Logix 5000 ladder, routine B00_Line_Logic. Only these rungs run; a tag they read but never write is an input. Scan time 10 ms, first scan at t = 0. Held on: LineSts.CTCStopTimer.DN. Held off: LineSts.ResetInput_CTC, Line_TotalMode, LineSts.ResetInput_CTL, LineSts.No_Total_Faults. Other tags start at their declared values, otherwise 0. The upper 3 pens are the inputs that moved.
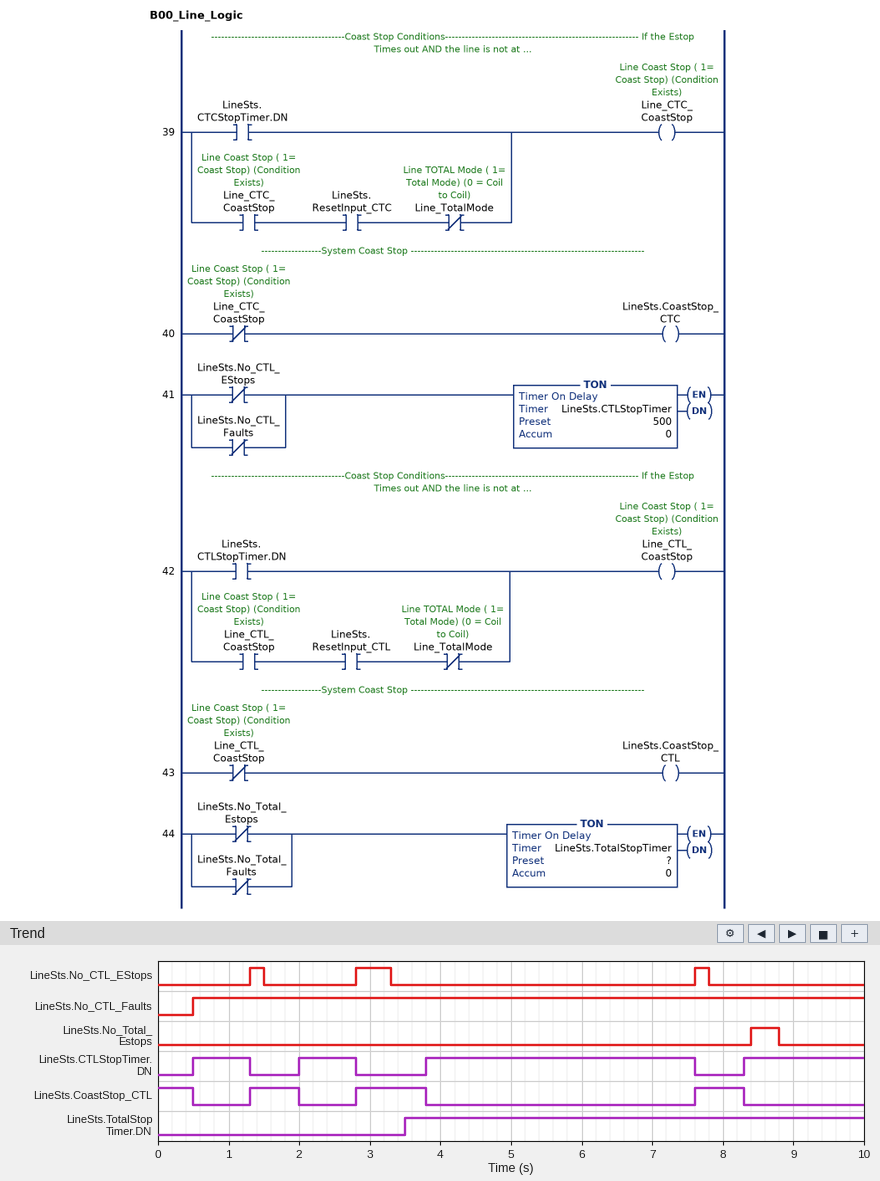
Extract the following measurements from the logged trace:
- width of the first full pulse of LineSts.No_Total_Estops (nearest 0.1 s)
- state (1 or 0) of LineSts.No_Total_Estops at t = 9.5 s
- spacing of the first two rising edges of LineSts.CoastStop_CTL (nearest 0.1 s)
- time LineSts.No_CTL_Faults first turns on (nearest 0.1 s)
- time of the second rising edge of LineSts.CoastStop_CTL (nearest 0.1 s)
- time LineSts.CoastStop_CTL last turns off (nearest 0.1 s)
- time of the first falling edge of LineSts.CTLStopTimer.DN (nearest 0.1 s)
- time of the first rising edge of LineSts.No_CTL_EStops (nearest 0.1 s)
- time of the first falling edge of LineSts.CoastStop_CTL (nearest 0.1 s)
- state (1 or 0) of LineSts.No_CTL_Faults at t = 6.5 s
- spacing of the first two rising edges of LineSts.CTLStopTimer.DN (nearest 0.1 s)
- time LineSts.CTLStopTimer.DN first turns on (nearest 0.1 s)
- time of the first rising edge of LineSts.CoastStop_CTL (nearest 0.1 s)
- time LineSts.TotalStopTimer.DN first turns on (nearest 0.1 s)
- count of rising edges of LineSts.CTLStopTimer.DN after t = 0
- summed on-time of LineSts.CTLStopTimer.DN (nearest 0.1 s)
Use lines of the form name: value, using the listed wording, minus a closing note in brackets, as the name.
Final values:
width of the first full pulse of LineSts.No_Total_Estops: 0.4 s
state (1 or 0) of LineSts.No_Total_Estops at t = 9.5 s: 0
spacing of the first two rising edges of LineSts.CoastStop_CTL: 1.5 s
time LineSts.No_CTL_Faults first turns on: 0.5 s
time of the second rising edge of LineSts.CoastStop_CTL: 2.8 s
time LineSts.CoastStop_CTL last turns off: 8.3 s
time of the first falling edge of LineSts.CTLStopTimer.DN: 1.3 s
time of the first rising edge of LineSts.No_CTL_EStops: 1.3 s
time of the first falling edge of LineSts.CoastStop_CTL: 0.5 s
state (1 or 0) of LineSts.No_CTL_Faults at t = 6.5 s: 1
spacing of the first two rising edges of LineSts.CTLStopTimer.DN: 1.5 s
time LineSts.CTLStopTimer.DN first turns on: 0.5 s
time of the first rising edge of LineSts.CoastStop_CTL: 1.3 s
time LineSts.TotalStopTimer.DN first turns on: 3.5 s
count of rising edges of LineSts.CTLStopTimer.DN after t = 0: 4
summed on-time of LineSts.CTLStopTimer.DN: 7.1 s
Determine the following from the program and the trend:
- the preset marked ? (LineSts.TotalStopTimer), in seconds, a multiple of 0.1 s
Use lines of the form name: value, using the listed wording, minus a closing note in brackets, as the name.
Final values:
the preset marked ? (LineSts.TotalStopTimer), in seconds, a multiple of 0.1 s: 3.5 s
